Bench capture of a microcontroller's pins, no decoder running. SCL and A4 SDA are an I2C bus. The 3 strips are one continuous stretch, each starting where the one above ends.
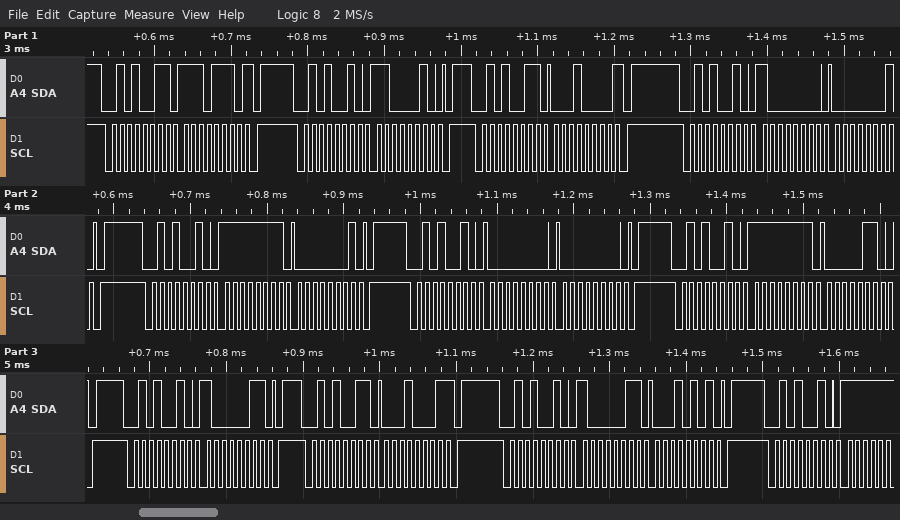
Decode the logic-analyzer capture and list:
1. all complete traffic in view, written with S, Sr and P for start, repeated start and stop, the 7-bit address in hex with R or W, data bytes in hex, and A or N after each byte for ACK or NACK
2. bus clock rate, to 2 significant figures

S 29R A EE N P S 29W A C2 A P S 29R A 10 N P S 29W A 80 A 01 A P S 29W A FF A 01 A P S 29W A 00 A 00 A P S 29W A FF A 06 A P S 29W A 83 A P S 29R A 11 N P S 29W A 83 A 15 A P S 29W A
100 kHz
